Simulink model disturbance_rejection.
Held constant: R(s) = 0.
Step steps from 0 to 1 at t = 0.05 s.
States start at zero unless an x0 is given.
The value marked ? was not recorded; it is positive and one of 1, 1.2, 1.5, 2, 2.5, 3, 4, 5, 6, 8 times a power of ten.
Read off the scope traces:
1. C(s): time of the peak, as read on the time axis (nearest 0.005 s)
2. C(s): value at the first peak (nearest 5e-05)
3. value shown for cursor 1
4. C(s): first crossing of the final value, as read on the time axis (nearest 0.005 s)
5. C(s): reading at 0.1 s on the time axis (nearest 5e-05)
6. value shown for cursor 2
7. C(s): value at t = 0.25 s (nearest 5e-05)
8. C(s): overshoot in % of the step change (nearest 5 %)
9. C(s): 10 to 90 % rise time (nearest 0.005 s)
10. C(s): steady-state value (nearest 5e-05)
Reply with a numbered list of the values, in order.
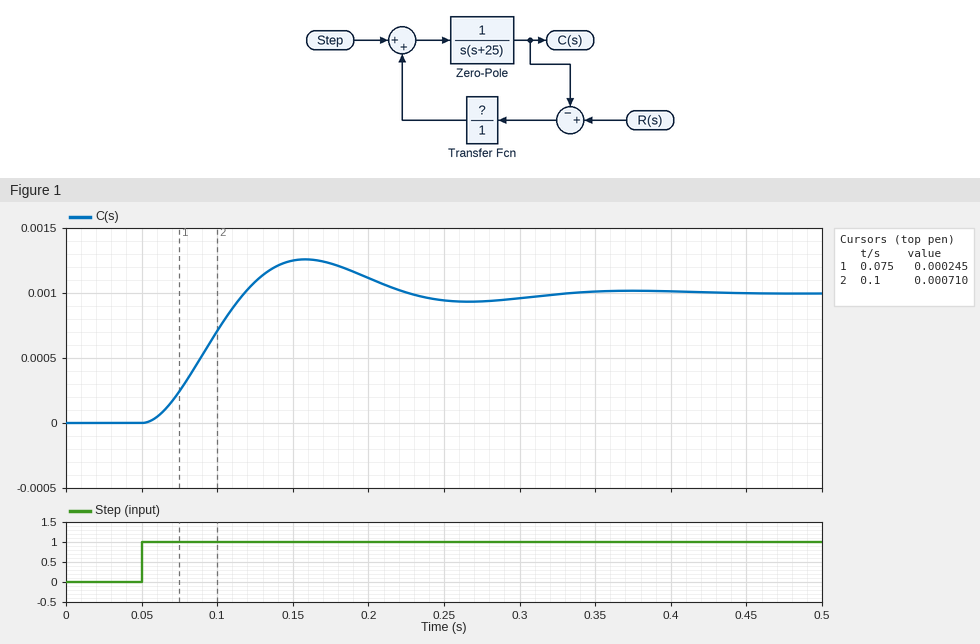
1. 0.160 s
2. 0.00125
3. 0.000245
4. 0.120 s
5. 0.00070
6. 0.000710
7. 0.00095
8. 25 %
9. 0.045 s
10. 0.00100
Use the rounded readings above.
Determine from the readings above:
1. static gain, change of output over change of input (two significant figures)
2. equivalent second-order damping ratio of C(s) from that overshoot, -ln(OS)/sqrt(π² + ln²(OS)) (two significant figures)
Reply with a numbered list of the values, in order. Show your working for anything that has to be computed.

1. (0.001 - 0) / (1 - 0) = 0.0010
2. ln(0.25) = -1.386; 1.386 / sqrt(9.870 + 1.922) = 0.40
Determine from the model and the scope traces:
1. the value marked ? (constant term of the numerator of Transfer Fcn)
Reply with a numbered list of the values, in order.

1. 1000
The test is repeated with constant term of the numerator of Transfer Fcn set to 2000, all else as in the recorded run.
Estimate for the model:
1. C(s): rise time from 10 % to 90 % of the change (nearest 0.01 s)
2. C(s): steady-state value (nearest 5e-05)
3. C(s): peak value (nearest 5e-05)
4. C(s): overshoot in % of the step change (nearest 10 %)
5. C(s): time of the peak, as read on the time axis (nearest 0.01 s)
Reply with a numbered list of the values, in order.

1. 0.03 s
2. 0.00050
3. 0.00070
4. 40 %
5. 0.12 s
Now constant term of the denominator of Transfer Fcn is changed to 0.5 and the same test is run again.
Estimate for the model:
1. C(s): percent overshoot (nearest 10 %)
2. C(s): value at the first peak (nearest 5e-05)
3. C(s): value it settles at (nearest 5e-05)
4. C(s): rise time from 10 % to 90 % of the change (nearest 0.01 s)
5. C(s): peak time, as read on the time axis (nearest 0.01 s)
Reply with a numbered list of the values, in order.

1. 40 %
2. 0.00070
3. 0.00050
4. 0.03 s
5. 0.12 s
